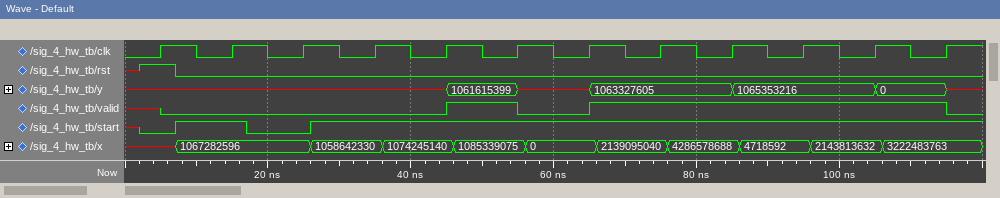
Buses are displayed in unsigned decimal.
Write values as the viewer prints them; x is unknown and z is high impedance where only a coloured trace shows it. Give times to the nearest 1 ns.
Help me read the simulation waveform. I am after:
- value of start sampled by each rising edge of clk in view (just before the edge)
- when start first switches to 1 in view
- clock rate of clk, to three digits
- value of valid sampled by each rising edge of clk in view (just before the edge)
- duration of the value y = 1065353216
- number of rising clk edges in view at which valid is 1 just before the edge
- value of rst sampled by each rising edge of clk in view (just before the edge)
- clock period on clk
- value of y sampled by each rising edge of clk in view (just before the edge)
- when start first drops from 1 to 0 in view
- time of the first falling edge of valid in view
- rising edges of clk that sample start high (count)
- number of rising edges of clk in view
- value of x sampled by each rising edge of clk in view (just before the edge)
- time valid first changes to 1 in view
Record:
0 1 0 1 1 1 1 1 1 1 1 1
7 ns
100 MHz
x 0 0 0 0 1 0 1 1 1 1 1
20 ns
6
1 0 0 0 0 0 0 0 0 0 0 0
10 ns
x, x, x, x, x, 1061615399, x, 1063327605, 1063327605, 1065353216, 1065353216, 0
17 ns
55 ns
10
12
x, 1067282596, 1067282596, 1058642330, 1074245140, 1085339075, 0, 2139095040, 4286578688, 4718592, 2143813632, 3222483763
45 ns
